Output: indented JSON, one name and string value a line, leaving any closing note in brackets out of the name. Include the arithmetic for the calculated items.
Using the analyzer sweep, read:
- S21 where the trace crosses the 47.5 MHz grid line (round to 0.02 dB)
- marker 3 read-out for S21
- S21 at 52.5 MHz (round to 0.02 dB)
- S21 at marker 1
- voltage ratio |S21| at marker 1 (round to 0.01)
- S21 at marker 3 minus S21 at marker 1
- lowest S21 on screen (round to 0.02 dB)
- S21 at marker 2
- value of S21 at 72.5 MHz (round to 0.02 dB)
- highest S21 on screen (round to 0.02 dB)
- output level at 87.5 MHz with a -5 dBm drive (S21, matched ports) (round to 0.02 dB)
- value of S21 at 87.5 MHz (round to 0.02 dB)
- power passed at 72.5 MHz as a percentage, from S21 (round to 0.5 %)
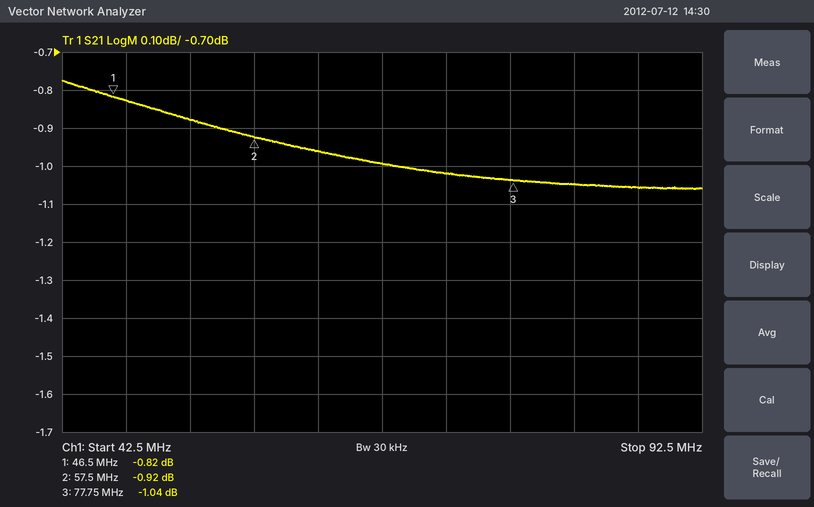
{
  "S21 where the trace crosses the 47.5 MHz grid line": "-0.82 dB",
  "marker 3 read-out for S21": "-1.04 dB",
  "S21 at 52.5 MHz": "-0.88 dB",
  "S21 at marker 1": "-0.82 dB",
  "voltage ratio |S21| at marker 1": "10^(-0.82/20) ≈ 0.91",
  "S21 at marker 3 minus S21 at marker 1": "-1.04 − (-0.82) = -0.22 dB",
  "lowest S21 on screen": "-1.06 dB",
  "S21 at marker 2": "-0.92 dB",
  "value of S21 at 72.5 MHz": "-1.02 dB",
  "highest S21 on screen": "-0.78 dB",
  "output level at 87.5 MHz with a -5 dBm drive (S21, matched ports)": "-5 dBm + (-1.06 dB) = -6.06 dBm",
  "value of S21 at 87.5 MHz": "-1.06 dB",
  "power passed at 72.5 MHz as a percentage, from S21": "10^(-1.02/10) ≈ 79.1 %, so 79.0 % to the nearest 0.5 %"
}
